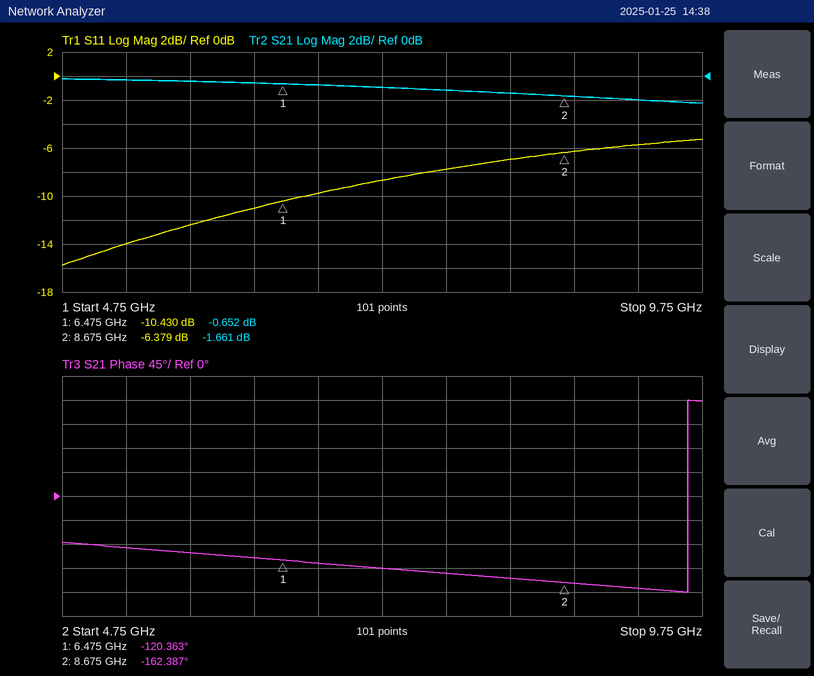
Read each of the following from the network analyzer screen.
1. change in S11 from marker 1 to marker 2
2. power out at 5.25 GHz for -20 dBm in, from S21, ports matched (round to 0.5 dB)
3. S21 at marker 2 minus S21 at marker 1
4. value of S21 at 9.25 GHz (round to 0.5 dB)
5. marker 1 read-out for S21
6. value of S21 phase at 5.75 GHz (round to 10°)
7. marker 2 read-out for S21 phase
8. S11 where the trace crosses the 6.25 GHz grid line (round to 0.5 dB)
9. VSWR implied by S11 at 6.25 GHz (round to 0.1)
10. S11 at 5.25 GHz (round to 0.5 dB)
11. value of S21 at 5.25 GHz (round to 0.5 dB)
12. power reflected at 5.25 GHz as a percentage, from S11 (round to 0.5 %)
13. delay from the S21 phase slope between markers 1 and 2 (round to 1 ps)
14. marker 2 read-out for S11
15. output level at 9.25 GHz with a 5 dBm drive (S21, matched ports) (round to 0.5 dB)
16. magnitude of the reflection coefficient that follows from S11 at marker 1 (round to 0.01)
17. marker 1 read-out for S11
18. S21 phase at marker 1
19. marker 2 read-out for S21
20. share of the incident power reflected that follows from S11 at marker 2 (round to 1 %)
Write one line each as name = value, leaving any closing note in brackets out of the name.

change in S11 from marker 1 to marker 2 = 4.051 dB
power out at 5.25 GHz for -20 dBm in, from S21, ports matched = -20.5 dBm
S21 at marker 2 minus S21 at marker 1 = -1.009 dB
value of S21 at 9.25 GHz = -2.0 dB
marker 1 read-out for S21 = -0.652 dB
value of S21 phase at 5.75 GHz = -110°
marker 2 read-out for S21 phase = -162.387°
S11 where the trace crosses the 6.25 GHz grid line = -11.0 dB
VSWR implied by S11 at 6.25 GHz = 1.8
S11 at 5.25 GHz = -14.0 dB
value of S21 at 5.25 GHz = -0.5 dB
power reflected at 5.25 GHz as a percentage, from S11 = 4.0 %
delay from the S21 phase slope between markers 1 and 2 = 53 ps
marker 2 read-out for S11 = -6.379 dB
output level at 9.25 GHz with a 5 dBm drive (S21, matched ports) = 3.0 dBm
magnitude of the reflection coefficient that follows from S11 at marker 1 = 0.30
marker 1 read-out for S11 = -10.430 dB
S21 phase at marker 1 = -120.363°
marker 2 read-out for S21 = -1.661 dB
share of the incident power reflected that follows from S11 at marker 2 = 23 %
